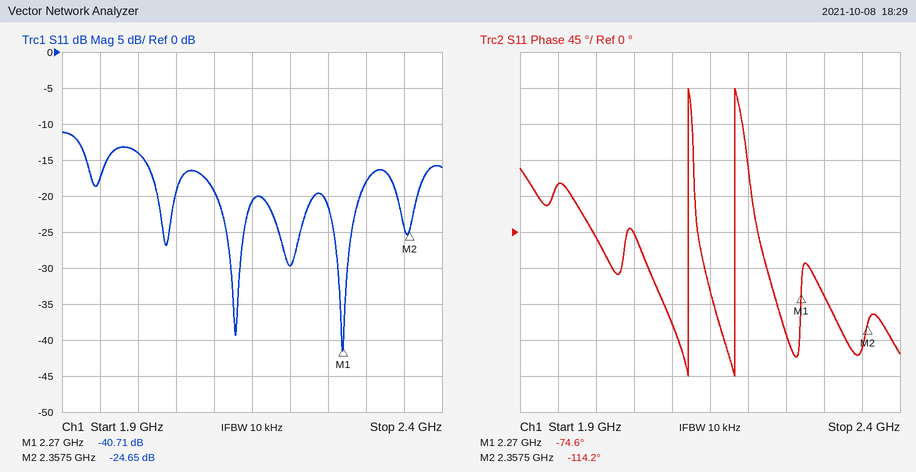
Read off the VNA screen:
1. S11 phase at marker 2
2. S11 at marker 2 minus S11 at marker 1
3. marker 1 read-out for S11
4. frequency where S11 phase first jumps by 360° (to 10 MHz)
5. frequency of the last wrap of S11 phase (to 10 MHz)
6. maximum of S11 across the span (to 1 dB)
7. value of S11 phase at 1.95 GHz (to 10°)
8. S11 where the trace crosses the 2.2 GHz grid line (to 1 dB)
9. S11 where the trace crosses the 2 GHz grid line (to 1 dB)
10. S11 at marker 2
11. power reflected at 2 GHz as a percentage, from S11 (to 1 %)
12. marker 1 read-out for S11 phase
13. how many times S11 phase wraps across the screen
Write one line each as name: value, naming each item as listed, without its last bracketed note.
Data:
S11 phase at marker 2: -114.2°
S11 at marker 2 minus S11 at marker 1: 16.06 dB
marker 1 read-out for S11: -40.71 dB
frequency where S11 phase first jumps by 360°: 2.12 GHz
frequency of the last wrap of S11 phase: 2.18 GHz
maximum of S11 across the span: -11 dB
value of S11 phase at 1.95 GHz: 60°
S11 where the trace crosses the 2.2 GHz grid line: -30 dB
S11 where the trace crosses the 2 GHz grid line: -14 dB
S11 at marker 2: -24.65 dB
power reflected at 2 GHz as a percentage, from S11: 4 %
marker 1 read-out for S11 phase: -74.6°
how many times S11 phase wraps across the screen: 2
